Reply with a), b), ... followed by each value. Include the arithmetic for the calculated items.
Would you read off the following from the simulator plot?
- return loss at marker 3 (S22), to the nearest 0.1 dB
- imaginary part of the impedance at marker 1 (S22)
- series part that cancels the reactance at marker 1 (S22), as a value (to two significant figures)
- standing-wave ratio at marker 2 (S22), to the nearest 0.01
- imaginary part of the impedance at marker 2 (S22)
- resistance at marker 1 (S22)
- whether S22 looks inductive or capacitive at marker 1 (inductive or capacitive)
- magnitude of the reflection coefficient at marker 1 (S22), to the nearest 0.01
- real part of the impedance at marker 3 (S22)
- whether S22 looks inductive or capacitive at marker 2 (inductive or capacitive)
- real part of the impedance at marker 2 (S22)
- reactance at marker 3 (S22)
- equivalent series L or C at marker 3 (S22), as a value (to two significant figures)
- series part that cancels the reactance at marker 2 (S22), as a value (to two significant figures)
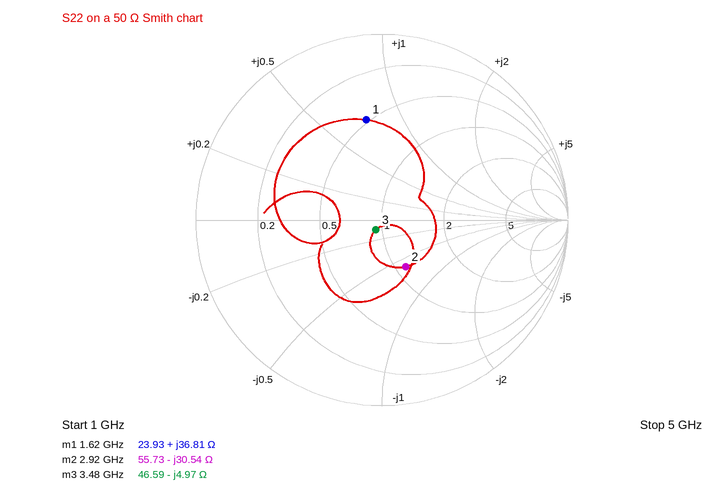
a) 24.1 dB
b) +36.81 Ω
c) C = 1/(2π × 1.62 GHz × 36.81 Ω) ≈ 2.7 pF
d) 1.79
e) -30.54 Ω
f) 23.93 Ω
g) inductive
h) 0.55
i) 46.59 Ω
j) capacitive
k) 55.73 Ω
l) -4.97 Ω
m) C = 1/(2π × 3.48 GHz × 4.97 Ω) ≈ 9.2 pF
n) L = 30.54 Ω/(2π × 2.92 GHz) ≈ 1.7 nH
